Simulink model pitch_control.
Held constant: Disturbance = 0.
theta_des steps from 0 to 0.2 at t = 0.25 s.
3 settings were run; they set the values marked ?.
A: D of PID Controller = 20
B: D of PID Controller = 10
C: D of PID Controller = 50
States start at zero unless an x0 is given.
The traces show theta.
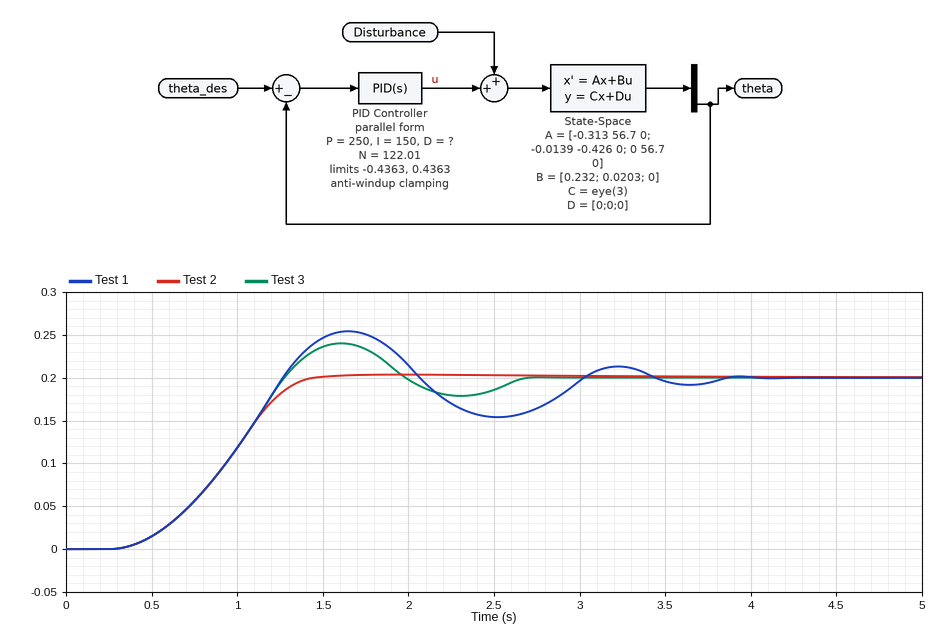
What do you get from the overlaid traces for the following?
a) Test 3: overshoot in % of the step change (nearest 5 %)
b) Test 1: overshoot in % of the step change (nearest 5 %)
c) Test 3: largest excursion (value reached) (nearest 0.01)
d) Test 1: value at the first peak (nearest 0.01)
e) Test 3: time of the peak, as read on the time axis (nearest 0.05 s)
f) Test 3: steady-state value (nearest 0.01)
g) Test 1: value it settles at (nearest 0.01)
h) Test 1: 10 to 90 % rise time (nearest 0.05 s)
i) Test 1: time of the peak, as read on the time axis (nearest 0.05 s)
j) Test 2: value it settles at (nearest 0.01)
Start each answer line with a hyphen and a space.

- 20 %
- 25 %
- 0.24
- 0.25
- 1.60 s
- 0.20
- 0.20
- 0.65 s
- 1.65 s
- 0.20
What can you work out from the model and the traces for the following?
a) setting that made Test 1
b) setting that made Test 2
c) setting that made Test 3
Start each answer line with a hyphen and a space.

- B
- C
- A
